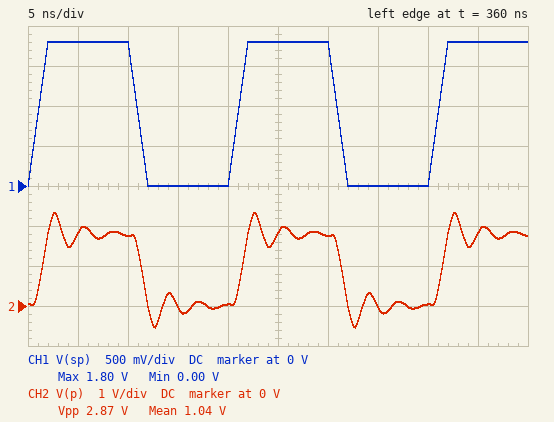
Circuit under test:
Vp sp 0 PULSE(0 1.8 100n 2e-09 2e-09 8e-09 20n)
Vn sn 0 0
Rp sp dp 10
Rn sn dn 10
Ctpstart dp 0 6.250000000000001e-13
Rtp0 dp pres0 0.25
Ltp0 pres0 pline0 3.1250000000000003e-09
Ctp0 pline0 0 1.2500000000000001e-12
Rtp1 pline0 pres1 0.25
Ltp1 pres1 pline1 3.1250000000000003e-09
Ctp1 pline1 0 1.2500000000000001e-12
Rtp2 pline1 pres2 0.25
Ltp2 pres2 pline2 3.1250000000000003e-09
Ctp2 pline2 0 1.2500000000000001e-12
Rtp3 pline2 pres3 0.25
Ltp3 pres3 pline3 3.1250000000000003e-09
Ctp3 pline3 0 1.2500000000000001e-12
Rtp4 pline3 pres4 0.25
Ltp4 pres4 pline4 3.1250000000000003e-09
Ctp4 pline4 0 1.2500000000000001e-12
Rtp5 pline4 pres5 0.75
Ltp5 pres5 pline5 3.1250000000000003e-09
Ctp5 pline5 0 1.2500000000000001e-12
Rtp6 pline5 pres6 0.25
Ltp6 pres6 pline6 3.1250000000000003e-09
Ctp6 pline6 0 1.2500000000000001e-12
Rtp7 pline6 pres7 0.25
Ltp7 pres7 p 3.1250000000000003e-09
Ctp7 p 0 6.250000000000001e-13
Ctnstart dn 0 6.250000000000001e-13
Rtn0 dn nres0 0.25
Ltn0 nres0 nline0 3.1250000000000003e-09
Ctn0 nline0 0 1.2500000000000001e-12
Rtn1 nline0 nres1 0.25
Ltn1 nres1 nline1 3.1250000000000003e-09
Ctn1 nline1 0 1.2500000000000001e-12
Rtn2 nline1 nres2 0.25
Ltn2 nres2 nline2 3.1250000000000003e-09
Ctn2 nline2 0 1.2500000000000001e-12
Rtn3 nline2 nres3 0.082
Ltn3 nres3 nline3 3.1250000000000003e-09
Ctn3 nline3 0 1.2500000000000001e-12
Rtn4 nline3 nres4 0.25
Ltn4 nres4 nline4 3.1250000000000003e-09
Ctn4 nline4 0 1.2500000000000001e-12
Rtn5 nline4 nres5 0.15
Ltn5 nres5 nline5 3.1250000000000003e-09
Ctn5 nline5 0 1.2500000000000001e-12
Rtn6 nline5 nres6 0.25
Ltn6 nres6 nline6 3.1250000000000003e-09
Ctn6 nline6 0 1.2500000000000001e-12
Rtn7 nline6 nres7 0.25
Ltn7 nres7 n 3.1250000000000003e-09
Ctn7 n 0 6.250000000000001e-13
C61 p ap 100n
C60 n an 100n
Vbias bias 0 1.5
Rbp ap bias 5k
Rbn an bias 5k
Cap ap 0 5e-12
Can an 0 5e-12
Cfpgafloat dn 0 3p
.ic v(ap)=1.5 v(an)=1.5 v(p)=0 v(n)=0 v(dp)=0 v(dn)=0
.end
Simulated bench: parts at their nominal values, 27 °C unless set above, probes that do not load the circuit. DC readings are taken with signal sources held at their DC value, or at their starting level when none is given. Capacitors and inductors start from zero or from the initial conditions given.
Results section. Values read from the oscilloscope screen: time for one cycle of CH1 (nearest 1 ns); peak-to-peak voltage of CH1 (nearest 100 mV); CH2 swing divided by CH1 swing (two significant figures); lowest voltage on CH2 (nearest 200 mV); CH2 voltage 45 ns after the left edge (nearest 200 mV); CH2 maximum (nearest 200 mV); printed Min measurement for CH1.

20 ns
1.8 V
1.6
-600 mV
1.8 V
2.4 V
0.00 V
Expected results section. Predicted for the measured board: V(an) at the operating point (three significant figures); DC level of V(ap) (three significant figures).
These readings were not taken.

1.50 V
1.50 V
